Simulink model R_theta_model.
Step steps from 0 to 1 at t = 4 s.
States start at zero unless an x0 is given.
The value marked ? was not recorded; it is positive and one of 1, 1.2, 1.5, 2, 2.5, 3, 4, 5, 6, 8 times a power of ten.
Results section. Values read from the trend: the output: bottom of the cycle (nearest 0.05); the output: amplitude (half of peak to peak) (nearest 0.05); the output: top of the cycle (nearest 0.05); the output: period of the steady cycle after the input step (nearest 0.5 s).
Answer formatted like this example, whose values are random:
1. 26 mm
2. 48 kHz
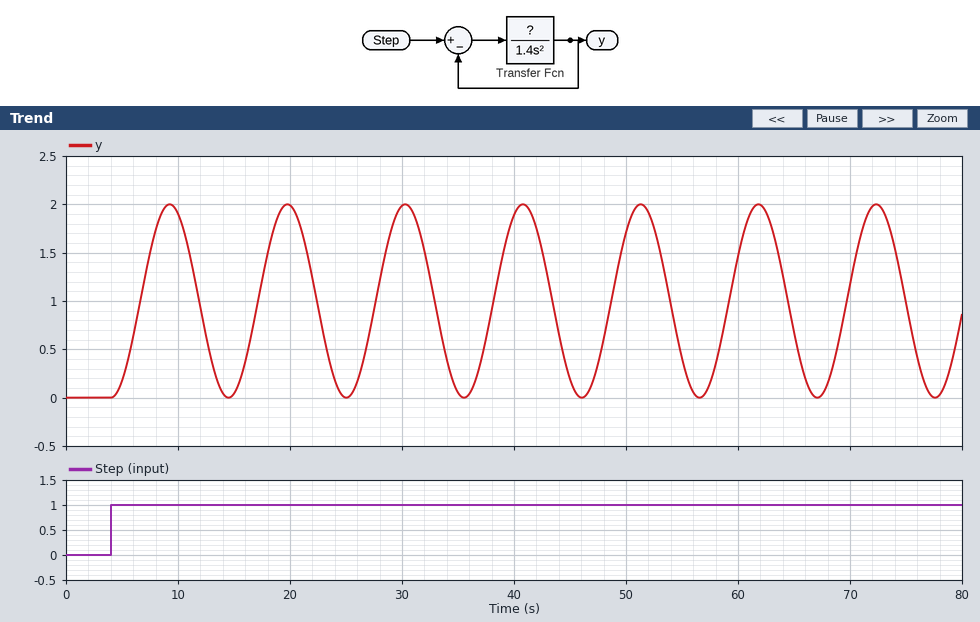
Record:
1. 0.00
2. 1.00
3. 2.00
4. 10.5 s
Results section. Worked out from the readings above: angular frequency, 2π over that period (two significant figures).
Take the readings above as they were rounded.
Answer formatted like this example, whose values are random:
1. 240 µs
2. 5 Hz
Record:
1. 0.60 rad/s
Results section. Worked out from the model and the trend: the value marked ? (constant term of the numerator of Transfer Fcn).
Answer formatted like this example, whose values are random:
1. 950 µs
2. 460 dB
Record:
1. 0.5
